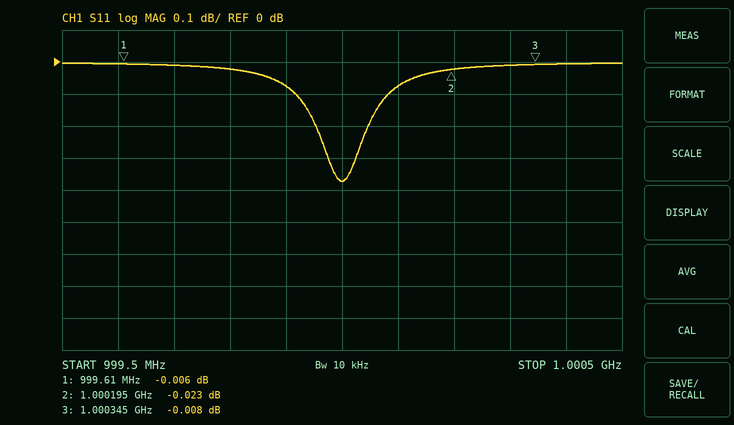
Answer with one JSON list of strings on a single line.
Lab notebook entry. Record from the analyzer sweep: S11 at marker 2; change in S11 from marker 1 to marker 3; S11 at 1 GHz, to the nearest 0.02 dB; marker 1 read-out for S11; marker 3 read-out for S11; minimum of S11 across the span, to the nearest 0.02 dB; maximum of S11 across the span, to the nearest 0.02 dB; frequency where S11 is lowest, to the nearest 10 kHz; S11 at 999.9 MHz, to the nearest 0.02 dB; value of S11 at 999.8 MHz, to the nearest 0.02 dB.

["-0.023 dB", "-0.002 dB", "-0.38 dB", "-0.006 dB", "-0.008 dB", "-0.38 dB", "0.00 dB", "1.00000 GHz", "-0.08 dB", "-0.02 dB"]
